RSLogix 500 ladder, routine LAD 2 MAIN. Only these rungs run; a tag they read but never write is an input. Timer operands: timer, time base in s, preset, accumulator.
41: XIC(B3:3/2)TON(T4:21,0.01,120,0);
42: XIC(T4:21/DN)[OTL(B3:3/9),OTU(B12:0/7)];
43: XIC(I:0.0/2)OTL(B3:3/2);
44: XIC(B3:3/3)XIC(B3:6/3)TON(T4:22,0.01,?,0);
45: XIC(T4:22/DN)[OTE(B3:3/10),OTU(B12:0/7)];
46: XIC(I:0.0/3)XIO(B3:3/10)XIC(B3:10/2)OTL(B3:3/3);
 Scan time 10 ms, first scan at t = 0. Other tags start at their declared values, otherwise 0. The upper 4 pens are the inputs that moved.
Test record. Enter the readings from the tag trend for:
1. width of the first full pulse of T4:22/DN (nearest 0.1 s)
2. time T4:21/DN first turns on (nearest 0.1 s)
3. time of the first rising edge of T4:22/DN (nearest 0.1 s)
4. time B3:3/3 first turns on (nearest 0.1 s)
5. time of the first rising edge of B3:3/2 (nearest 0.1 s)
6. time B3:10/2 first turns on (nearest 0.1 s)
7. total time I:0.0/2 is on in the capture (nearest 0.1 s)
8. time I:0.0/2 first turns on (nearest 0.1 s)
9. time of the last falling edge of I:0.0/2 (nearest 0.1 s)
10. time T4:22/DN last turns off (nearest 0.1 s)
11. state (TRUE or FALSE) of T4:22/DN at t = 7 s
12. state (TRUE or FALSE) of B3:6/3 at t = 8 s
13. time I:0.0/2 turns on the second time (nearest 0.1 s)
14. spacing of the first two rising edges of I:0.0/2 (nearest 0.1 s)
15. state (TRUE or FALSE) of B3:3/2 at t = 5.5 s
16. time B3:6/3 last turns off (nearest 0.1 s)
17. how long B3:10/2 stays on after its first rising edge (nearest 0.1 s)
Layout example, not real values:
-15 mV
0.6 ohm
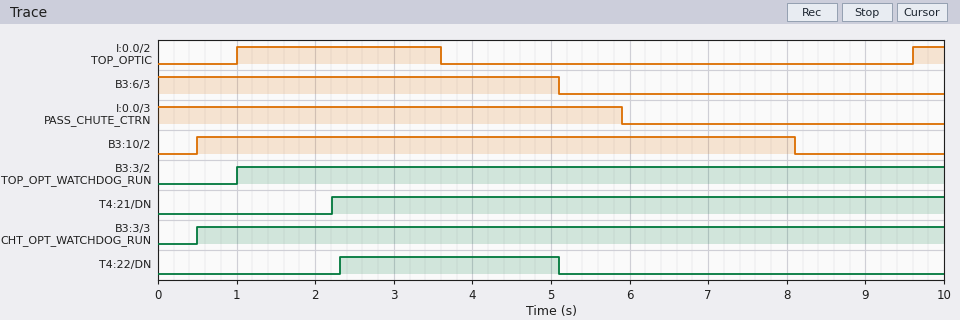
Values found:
2.8 s
2.2 s
2.3 s
0.5 s
1.0 s
0.5 s
3.0 s
1.0 s
3.6 s
5.1 s
FALSE
FALSE
9.6 s
8.6 s
TRUE
5.1 s
7.6 s
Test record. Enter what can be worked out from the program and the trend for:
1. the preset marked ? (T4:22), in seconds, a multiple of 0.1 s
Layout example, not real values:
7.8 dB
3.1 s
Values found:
1.8 s
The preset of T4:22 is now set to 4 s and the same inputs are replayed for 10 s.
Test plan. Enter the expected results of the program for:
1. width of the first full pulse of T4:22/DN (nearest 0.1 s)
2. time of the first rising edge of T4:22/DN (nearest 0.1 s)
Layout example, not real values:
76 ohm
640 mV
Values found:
0.6 s
4.5 s
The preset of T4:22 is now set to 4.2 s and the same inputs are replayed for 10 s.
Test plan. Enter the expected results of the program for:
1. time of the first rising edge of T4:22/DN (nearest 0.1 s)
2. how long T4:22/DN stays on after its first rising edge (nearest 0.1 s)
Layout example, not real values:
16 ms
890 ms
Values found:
4.7 s
0.4 s
